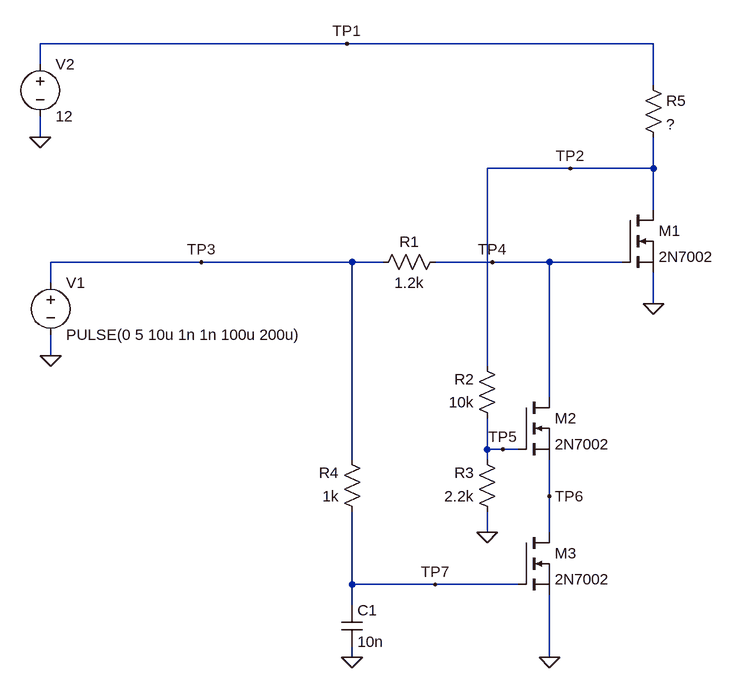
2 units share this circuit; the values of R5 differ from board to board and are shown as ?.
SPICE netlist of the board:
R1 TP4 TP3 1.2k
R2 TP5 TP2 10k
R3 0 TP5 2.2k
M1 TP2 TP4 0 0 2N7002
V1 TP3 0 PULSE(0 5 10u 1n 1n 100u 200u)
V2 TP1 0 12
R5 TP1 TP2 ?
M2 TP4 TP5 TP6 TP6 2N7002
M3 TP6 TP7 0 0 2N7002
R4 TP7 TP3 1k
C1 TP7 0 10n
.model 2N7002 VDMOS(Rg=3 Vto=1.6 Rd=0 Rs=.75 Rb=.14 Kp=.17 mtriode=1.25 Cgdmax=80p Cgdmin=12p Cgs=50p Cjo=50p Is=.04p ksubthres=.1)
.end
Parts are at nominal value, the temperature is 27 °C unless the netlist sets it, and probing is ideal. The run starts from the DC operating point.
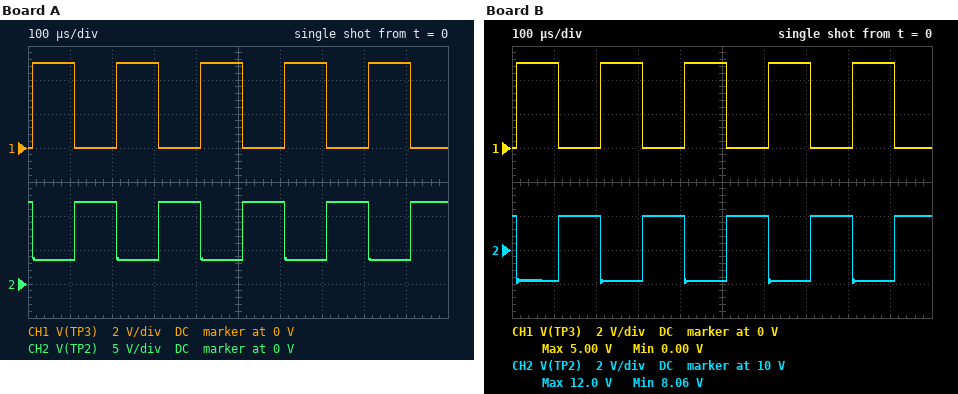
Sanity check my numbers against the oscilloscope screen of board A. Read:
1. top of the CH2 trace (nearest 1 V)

12 V
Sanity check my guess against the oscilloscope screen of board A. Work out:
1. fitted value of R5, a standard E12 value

12 Ω
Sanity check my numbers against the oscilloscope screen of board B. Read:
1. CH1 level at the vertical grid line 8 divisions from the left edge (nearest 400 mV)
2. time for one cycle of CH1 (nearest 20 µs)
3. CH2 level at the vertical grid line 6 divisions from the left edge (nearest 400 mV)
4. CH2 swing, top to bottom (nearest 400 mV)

0 V
200 µs
12.0 V
4.0 V
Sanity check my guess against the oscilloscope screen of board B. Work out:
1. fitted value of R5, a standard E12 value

5.6 Ω
